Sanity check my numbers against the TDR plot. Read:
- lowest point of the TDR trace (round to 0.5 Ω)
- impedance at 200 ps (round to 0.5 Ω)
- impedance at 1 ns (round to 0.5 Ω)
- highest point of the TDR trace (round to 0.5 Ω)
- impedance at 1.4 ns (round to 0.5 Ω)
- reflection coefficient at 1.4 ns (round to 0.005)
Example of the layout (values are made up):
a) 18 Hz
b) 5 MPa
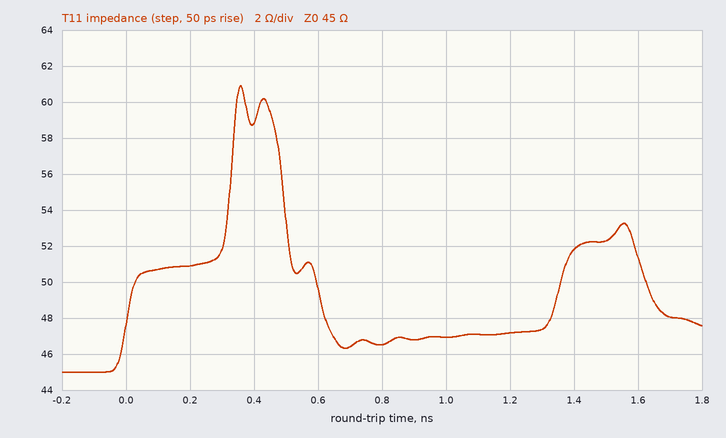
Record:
a) 45.0 Ω
b) 51.0 Ω
c) 47.0 Ω
d) 61.0 Ω
e) 52.0 Ω
f) +0.070
